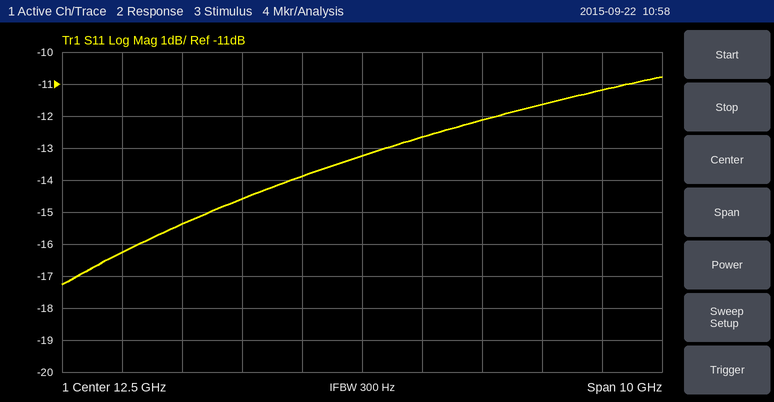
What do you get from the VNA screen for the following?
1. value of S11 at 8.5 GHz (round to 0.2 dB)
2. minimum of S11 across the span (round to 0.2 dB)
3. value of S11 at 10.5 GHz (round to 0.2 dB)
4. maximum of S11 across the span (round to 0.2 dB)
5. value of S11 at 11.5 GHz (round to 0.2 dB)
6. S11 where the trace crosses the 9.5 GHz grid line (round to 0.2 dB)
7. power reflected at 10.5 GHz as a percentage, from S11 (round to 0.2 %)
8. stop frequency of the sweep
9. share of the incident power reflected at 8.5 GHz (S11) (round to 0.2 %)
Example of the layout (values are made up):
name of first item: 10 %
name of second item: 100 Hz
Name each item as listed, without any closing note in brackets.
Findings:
value of S11 at 8.5 GHz: -16.2 dB
minimum of S11 across the span: -17.2 dB
value of S11 at 10.5 GHz: -14.6 dB
maximum of S11 across the span: -10.8 dB
value of S11 at 11.5 GHz: -13.8 dB
S11 where the trace crosses the 9.5 GHz grid line: -15.4 dB
power reflected at 10.5 GHz as a percentage, from S11: 3.4 %
stop frequency of the sweep: 17.5 GHz
share of the incident power reflected at 8.5 GHz (S11): 2.4 %
